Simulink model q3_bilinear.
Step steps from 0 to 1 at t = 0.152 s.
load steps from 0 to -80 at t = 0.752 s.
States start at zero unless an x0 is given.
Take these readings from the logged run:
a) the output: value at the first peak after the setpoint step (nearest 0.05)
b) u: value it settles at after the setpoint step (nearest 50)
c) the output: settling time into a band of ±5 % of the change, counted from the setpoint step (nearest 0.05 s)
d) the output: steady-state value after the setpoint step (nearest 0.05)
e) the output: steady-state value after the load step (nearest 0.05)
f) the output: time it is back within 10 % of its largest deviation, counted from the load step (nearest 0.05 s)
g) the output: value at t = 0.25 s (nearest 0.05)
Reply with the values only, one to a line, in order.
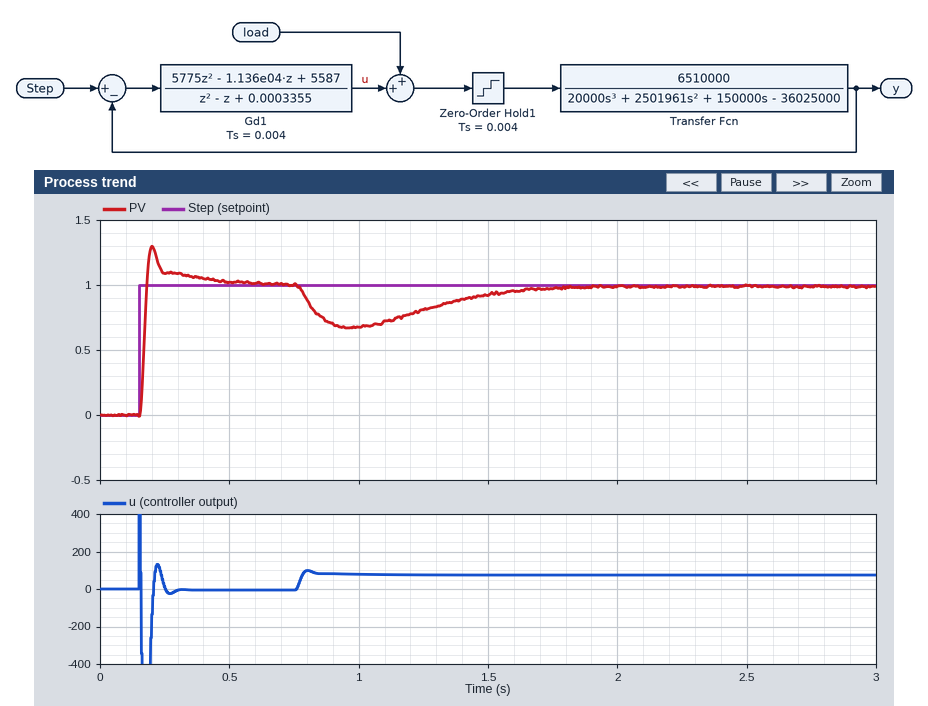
1.30
0
0.25 s
1.00
1.00
0.85 s
1.10
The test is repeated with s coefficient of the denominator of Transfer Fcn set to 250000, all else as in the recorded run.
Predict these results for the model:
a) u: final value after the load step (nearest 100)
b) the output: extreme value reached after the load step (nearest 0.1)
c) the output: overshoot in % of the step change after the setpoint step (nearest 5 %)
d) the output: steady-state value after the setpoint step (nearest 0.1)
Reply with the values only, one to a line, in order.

100
0.7
30 %
1.0
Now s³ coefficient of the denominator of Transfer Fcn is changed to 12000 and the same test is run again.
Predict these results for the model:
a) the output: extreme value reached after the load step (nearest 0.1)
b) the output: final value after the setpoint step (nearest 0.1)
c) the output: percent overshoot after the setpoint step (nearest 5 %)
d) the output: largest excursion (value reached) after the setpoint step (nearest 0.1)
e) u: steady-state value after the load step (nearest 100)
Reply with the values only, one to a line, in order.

0.7
1.0
20 %
1.2
100
